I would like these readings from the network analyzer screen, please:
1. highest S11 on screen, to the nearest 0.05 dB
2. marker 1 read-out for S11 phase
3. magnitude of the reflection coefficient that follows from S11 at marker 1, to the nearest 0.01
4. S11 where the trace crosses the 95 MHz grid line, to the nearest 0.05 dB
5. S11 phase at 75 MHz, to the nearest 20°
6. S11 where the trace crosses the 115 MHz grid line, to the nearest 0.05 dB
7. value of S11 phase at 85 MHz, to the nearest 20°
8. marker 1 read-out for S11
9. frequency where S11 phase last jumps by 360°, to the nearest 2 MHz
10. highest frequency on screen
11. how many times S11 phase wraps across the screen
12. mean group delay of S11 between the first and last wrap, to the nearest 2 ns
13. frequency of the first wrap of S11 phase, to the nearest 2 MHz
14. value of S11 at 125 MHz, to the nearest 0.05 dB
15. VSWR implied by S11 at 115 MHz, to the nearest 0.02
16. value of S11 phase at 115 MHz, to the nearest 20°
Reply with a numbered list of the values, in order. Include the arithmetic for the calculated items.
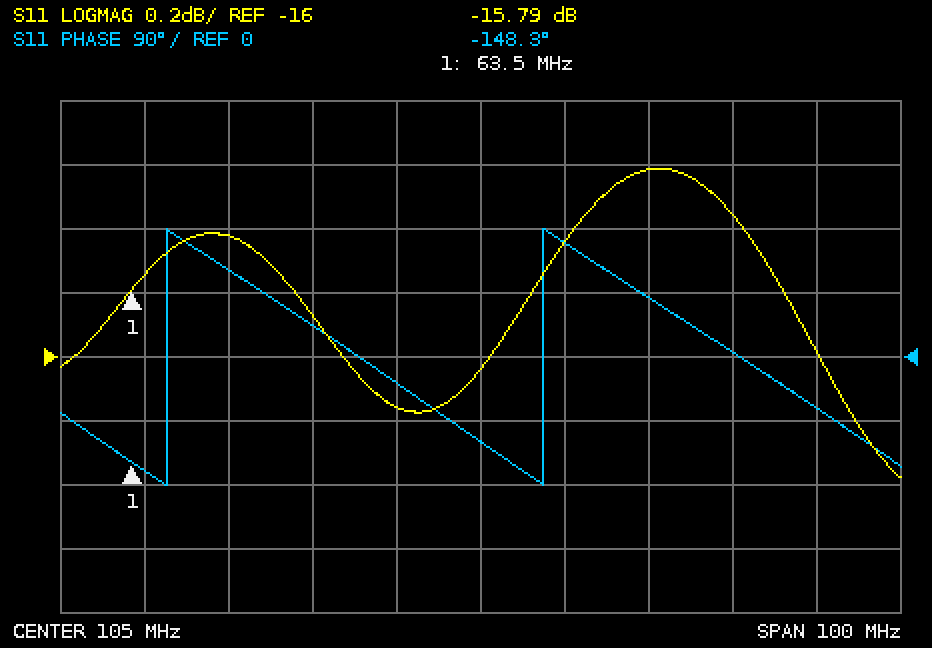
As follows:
1. -15.40 dB
2. -148.3°
3. 10^(-15.79/20) ≈ 0.16
4. -16.15 dB
5. 120°
6. -15.65 dB
7. 40°
8. -15.79 dB
9. 112 MHz
10. 155 MHz
11. 2
12. 1 cycle / (112 MHz − 68 MHz) ≈ 22.7 ns, so 22 ns to the nearest 2 ns
13. 68 MHz
14. -15.40 dB
15. |Γ| = 10^(-15.65/20) = 0.1650; VSWR = (1 + 0.1650)/(1 − 0.1650) ≈ 1.40
16. 160°
